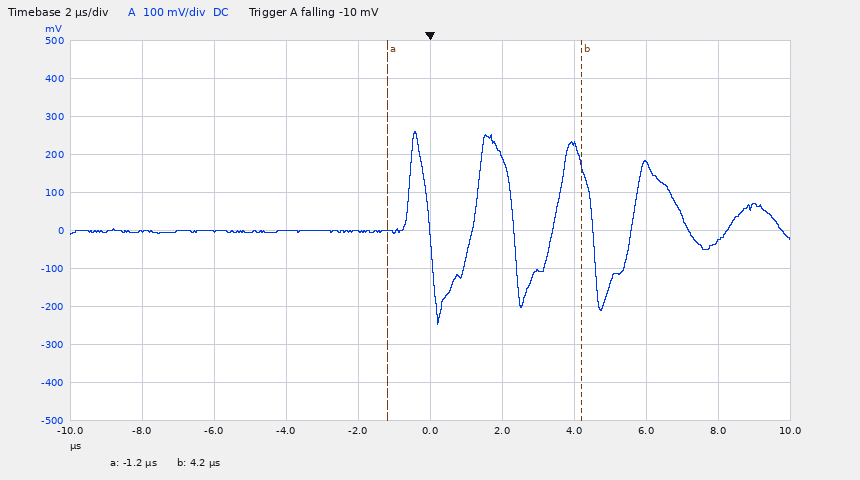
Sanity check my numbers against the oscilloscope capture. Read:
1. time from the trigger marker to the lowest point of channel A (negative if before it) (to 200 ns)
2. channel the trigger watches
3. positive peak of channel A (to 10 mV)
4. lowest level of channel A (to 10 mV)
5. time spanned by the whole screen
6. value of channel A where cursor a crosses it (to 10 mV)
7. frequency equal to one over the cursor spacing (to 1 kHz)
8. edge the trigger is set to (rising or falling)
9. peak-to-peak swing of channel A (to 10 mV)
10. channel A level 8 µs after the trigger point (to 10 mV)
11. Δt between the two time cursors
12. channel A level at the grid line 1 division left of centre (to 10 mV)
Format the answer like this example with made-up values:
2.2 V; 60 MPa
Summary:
+200 ns; channel A; 260 mV; -250 mV; 20 µs; 0 mV; 185 kHz; falling; 510 mV; -30 mV; 5.4 µs; 0 mV
